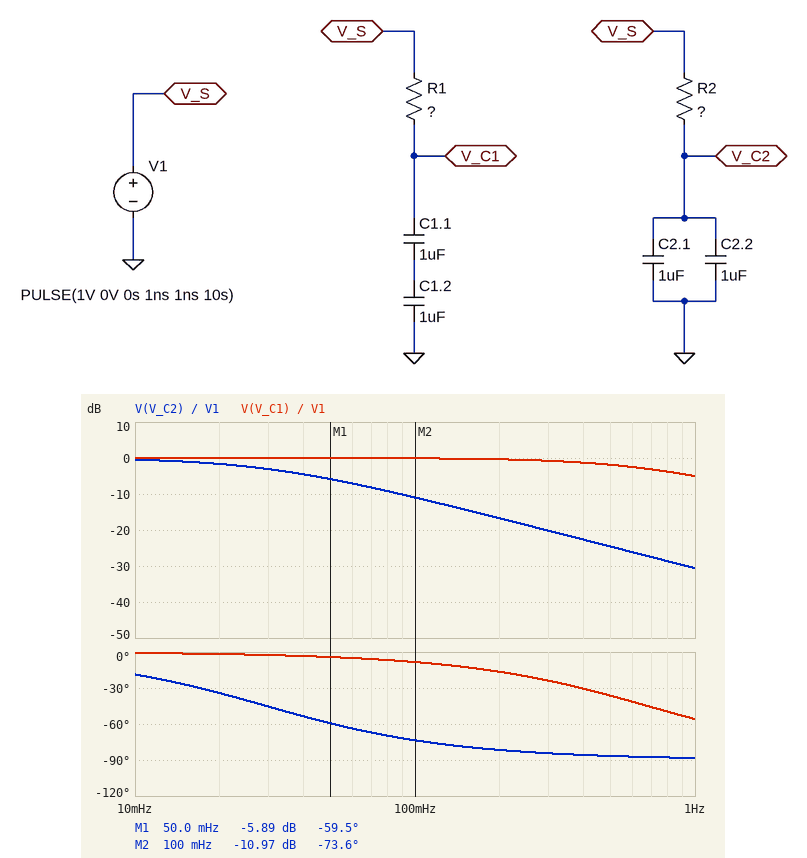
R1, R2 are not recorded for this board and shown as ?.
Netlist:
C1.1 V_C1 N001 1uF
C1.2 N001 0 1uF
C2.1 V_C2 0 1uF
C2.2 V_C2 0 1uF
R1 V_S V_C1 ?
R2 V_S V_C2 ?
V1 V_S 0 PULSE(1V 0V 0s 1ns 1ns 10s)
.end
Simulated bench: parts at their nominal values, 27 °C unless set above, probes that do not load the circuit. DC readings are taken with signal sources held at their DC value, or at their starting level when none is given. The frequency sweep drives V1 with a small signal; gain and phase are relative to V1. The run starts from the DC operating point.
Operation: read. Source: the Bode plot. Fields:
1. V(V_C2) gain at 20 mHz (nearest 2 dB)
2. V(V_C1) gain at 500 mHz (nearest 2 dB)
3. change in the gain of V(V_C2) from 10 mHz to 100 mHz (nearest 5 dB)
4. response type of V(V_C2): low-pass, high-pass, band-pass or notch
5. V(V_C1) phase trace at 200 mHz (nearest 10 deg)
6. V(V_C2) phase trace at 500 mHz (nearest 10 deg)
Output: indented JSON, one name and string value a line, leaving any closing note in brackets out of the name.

{
  "V(V_C2) gain at 20 mHz": "-2 dB",
  "V(V_C1) gain at 500 mHz": "-2 dB",
  "change in the gain of V(V_C2) from 10 mHz to 100 mHz": "-10 dB",
  "response type of V(V_C2): low-pass, high-pass, band-pass or notch": "low-pass",
  "V(V_C1) phase trace at 200 mHz": "-20 deg",
  "V(V_C2) phase trace at 500 mHz": "-90 deg"
}
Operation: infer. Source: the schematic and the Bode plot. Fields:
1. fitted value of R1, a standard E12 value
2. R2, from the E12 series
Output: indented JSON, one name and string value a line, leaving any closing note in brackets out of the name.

{
  "fitted value of R1, a standard E12 value": "470 kΩ",
  "R2, from the E12 series": "2.7 MΩ"
}
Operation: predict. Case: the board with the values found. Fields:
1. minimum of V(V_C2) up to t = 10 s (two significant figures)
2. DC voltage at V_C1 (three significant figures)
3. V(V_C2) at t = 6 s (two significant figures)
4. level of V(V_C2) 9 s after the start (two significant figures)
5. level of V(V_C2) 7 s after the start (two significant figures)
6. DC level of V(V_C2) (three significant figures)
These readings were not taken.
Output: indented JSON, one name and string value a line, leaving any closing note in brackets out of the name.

{
  "minimum of V(V_C2) up to t = 10 s": "160 mV",
  "DC voltage at V_C1": "1.00 V",
  "V(V_C2) at t = 6 s": "330 mV",
  "level of V(V_C2) 9 s after the start": "190 mV",
  "level of V(V_C2) 7 s after the start": "270 mV",
  "DC level of V(V_C2)": "1.00 V"
}
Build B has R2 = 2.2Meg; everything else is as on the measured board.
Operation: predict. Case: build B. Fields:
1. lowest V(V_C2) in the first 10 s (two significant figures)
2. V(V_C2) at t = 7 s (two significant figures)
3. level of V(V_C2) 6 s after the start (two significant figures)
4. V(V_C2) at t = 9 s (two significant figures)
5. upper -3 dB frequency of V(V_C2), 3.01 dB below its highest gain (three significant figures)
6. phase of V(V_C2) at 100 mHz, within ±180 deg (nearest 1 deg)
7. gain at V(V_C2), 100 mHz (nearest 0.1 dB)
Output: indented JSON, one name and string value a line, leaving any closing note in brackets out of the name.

{
  "lowest V(V_C2) in the first 10 s": "100 mV",
  "V(V_C2) at t = 7 s": "200 mV",
  "level of V(V_C2) 6 s after the start": "260 mV",
  "V(V_C2) at t = 9 s": "130 mV",
  "upper -3 dB frequency of V(V_C2), 3.01 dB below its highest gain": "36.2 mHz",
  "phase of V(V_C2) at 100 mHz, within ±180 deg": "-70 deg",
  "gain at V(V_C2), 100 mHz": "-9.4 dB"
}
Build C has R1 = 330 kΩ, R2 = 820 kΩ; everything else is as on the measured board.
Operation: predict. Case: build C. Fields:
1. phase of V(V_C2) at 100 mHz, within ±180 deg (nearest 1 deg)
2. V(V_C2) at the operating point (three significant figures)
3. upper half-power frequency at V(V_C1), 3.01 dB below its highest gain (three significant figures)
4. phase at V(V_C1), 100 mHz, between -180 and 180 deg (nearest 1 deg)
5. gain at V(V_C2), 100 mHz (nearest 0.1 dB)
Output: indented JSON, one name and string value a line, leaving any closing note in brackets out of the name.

{
  "phase of V(V_C2) at 100 mHz, within ±180 deg": "-46 deg",
  "V(V_C2) at the operating point": "1.00 V",
  "upper half-power frequency at V(V_C1), 3.01 dB below its highest gain": "965 mHz",
  "phase at V(V_C1), 100 mHz, between -180 and 180 deg": "-6 deg",
  "gain at V(V_C2), 100 mHz": "-3.1 dB"
}
